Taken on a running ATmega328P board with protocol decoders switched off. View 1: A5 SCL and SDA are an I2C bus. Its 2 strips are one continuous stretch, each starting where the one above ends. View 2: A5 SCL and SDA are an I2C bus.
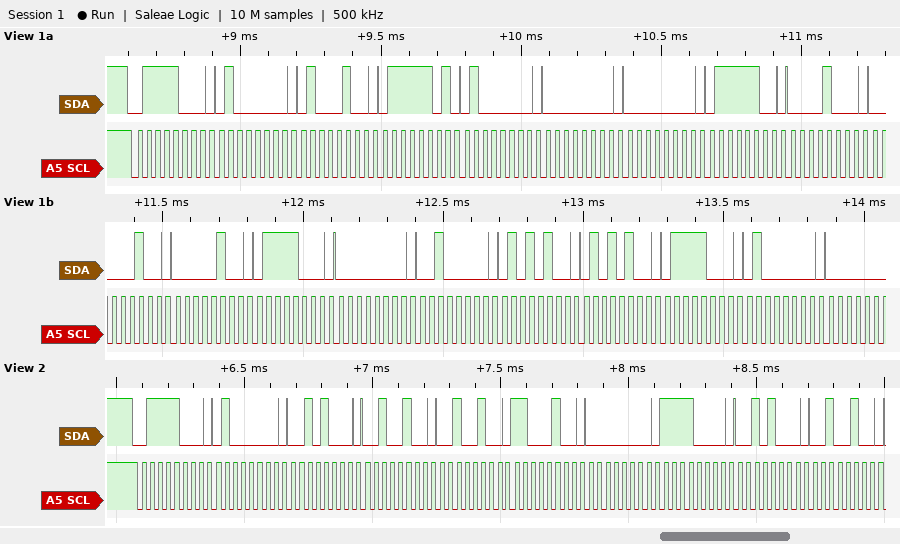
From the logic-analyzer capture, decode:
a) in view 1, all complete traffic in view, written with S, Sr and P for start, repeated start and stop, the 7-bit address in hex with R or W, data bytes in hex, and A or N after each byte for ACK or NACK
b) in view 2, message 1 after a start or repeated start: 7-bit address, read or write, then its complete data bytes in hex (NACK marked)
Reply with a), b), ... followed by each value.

a) S 3CW A 40 A 44 A 7D A 40 A 00 A 00 A 7C A 08 A 04 A 04 A 78 A 00 A 20 A 54 A 54 A 78 A 40 A
b) 0x3C write: 40 28 24 24 C4 00 F0 28 24
